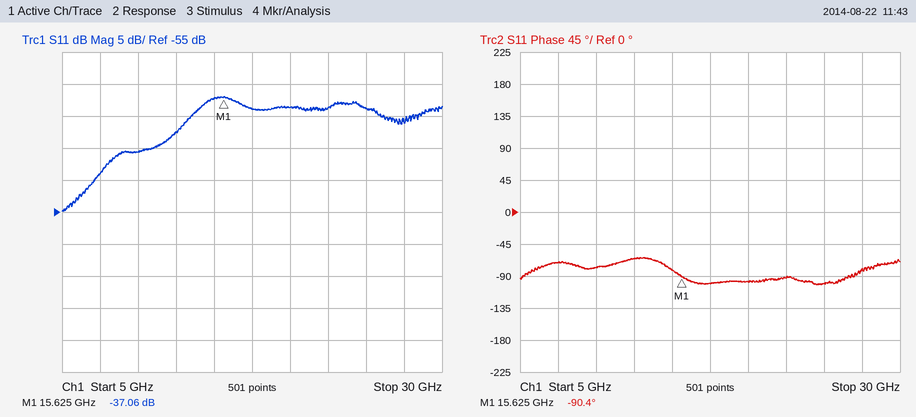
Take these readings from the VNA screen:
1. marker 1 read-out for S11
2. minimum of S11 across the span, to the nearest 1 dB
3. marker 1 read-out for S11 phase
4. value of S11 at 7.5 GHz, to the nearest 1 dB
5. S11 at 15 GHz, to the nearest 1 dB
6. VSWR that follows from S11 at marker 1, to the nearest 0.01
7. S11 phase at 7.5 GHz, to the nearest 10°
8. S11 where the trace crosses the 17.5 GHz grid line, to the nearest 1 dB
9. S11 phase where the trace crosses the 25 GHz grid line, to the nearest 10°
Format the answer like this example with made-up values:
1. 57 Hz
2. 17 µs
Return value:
1. -37.06 dB
2. -55 dB
3. -90.4°
4. -49 dB
5. -37 dB
6. 1.03
7. -70°
8. -39 dB
9. -100°
